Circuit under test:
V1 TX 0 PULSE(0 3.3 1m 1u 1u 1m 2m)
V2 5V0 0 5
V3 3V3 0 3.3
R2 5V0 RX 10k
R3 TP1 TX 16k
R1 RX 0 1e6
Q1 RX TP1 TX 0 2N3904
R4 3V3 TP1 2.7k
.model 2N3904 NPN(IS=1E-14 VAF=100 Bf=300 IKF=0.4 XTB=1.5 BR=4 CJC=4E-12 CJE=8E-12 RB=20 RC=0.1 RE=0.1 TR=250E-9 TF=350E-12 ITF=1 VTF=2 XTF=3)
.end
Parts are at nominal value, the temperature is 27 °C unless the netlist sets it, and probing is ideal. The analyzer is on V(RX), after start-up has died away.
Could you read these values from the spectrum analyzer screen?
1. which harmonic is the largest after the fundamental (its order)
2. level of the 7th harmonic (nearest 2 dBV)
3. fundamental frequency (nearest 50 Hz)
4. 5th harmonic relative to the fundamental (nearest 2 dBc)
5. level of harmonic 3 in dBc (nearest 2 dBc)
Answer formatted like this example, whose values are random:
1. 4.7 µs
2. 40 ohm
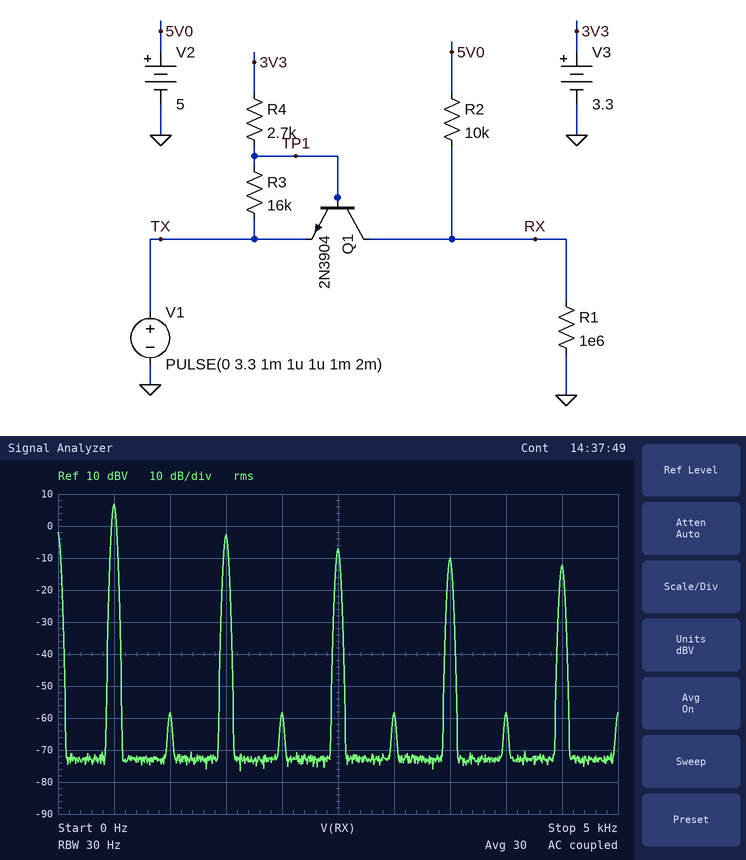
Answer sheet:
1. 3
2. -10 dBV
3. 500 Hz
4. -14 dBc
5. -10 dBc
